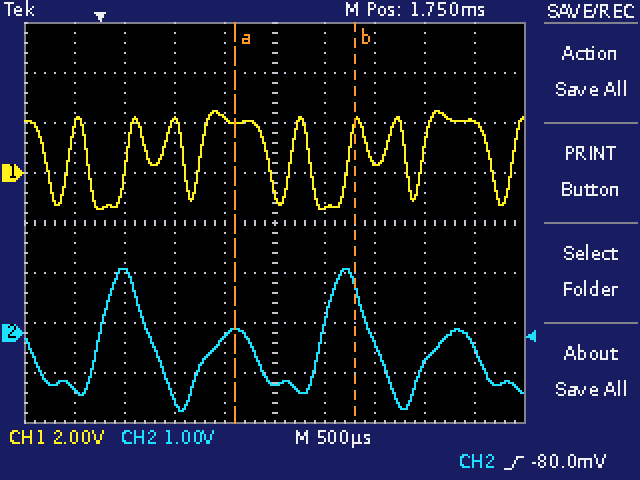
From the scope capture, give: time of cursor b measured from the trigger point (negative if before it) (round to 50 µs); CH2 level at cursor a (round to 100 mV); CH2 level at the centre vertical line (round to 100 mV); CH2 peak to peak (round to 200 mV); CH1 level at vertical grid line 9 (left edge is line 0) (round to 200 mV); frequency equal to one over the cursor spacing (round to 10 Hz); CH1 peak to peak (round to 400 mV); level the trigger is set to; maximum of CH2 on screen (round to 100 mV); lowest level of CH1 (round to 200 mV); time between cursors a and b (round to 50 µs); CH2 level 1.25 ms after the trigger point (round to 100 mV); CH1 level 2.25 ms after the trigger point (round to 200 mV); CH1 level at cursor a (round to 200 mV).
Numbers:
+2.55 ms
0.0 V
-1.0 V
2.8 V
2.0 V
830 Hz
4.0 V
-80.0 mV
1.3 V
-1.4 V
1.20 ms
-100 mV
-1.4 V
2.0 V
